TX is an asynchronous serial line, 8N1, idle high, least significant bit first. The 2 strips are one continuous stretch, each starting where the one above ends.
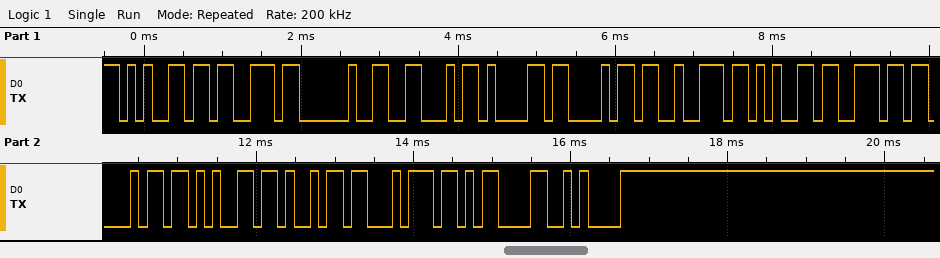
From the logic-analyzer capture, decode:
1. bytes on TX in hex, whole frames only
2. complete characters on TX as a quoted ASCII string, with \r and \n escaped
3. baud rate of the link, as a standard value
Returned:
0x65 0x73 0x20 0x46 0x61 0x68 0x72 0x65 0x6E 0x68 0x65 0x69 0x74 0x0D 0x0A
"es Fahrenheit\r\n"
9600 baud
